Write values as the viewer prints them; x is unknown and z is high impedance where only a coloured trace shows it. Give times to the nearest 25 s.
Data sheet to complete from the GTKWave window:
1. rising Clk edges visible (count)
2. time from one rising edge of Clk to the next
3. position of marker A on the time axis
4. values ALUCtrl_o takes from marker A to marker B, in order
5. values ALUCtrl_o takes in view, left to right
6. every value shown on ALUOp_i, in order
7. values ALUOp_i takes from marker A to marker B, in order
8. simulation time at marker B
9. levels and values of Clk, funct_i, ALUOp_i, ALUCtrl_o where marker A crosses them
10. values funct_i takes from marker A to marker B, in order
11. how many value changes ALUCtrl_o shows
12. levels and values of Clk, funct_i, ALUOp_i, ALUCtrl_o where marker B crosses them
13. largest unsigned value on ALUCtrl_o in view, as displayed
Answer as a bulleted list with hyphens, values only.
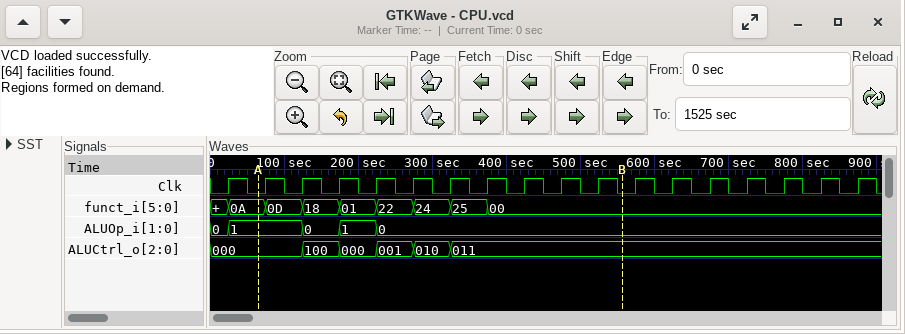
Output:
- 18
- 50 s
- 75 s
- 000, 100, 000, 001, 010, 011
- 000, 100, 000, 001, 010, 011
- 0, 1, 0, 1, 0
- 1, 0, 1, 0
- 550 s
- Clk=0, funct_i=0A, ALUOp_i=1, ALUCtrl_o=000
- 0A, 0D, 18, 01, 22, 24, 25, 00
- 5
- Clk=0, funct_i=00, ALUOp_i=0, ALUCtrl_o=011
- 100
